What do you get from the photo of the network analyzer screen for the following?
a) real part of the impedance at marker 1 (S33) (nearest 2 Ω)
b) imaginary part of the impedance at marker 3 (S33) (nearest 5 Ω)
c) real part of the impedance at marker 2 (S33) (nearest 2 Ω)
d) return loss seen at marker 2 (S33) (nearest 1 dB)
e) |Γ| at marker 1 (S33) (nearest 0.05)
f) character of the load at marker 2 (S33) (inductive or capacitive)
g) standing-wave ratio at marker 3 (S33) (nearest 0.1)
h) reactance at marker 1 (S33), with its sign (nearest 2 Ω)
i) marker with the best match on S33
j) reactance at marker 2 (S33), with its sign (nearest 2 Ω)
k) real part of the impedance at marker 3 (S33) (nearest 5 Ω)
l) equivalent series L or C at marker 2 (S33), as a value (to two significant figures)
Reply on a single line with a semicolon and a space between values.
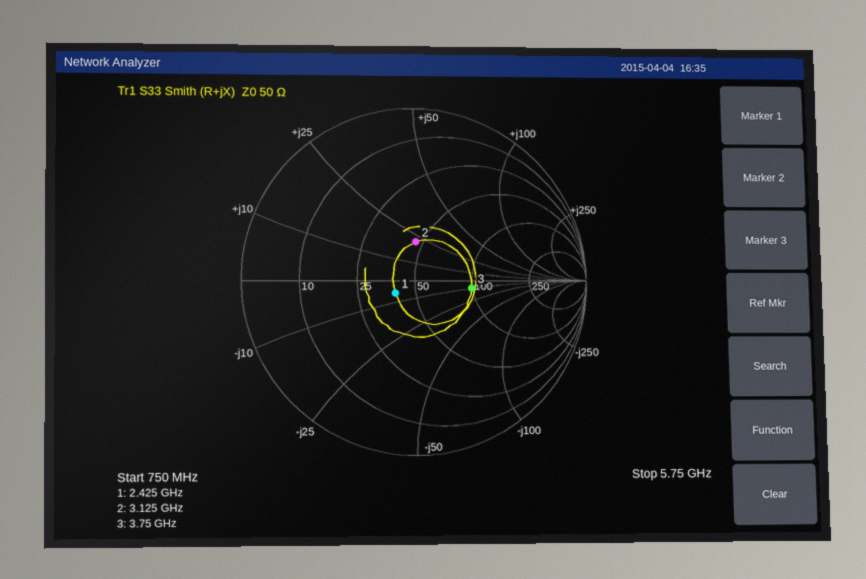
40 Ω; -10 Ω; 46 Ω; 13 dB; 0.15; inductive; 2.0; -6 Ω; marker 1; +22 Ω; 100 Ω; 1.1 nH
